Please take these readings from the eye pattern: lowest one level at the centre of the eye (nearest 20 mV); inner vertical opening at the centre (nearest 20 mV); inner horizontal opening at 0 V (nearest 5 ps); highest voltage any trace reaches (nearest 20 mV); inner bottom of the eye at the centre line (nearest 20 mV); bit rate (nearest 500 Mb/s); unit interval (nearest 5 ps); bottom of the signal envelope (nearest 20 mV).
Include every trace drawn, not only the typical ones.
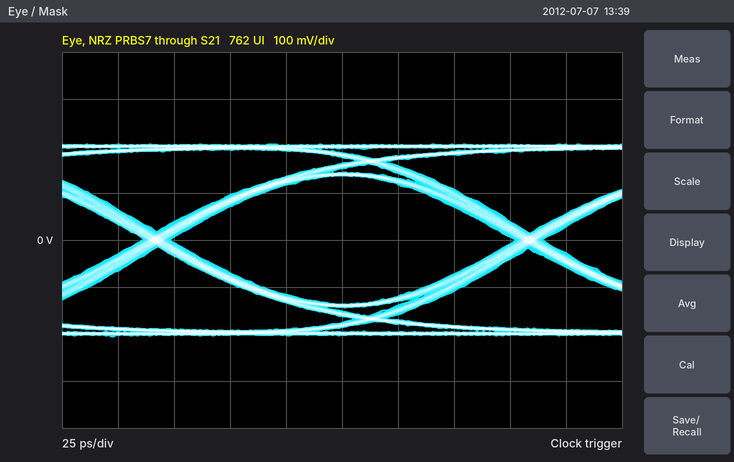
140 mV
280 mV
155 ps
200 mV
-140 mV
6.0 Gb/s
165 ps
-200 mV
